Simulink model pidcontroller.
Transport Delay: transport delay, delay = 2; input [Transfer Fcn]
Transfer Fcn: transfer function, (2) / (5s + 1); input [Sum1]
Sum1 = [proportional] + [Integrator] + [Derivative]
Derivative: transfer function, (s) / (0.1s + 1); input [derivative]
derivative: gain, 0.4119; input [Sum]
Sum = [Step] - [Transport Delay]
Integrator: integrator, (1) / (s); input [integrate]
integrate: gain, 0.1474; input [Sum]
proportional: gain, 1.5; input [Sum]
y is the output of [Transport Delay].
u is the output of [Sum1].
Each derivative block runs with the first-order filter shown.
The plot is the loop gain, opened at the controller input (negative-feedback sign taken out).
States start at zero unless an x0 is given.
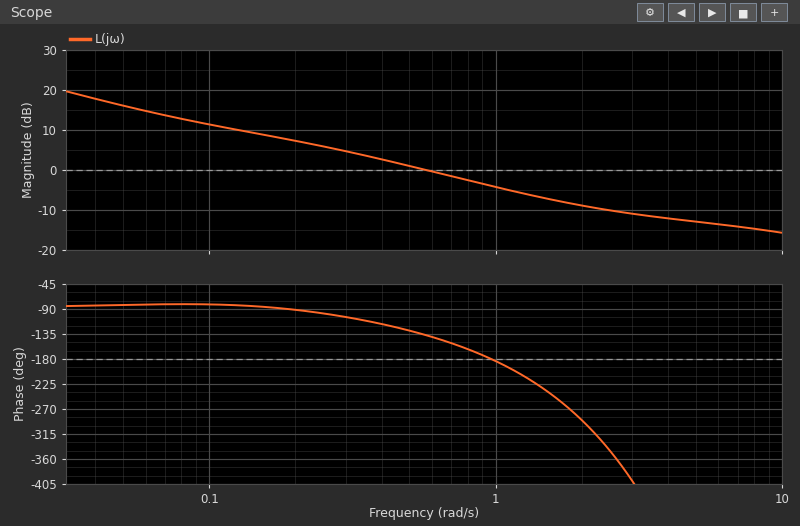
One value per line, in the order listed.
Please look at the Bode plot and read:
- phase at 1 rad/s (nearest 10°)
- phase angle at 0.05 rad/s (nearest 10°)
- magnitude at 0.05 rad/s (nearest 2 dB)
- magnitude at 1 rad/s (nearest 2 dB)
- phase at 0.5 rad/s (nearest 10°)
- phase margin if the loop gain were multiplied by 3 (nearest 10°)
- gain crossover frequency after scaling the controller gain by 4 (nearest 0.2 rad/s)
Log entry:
-180°
-80°
16 dB
-4 dB
-130°
-140°
4.0 rad/s
